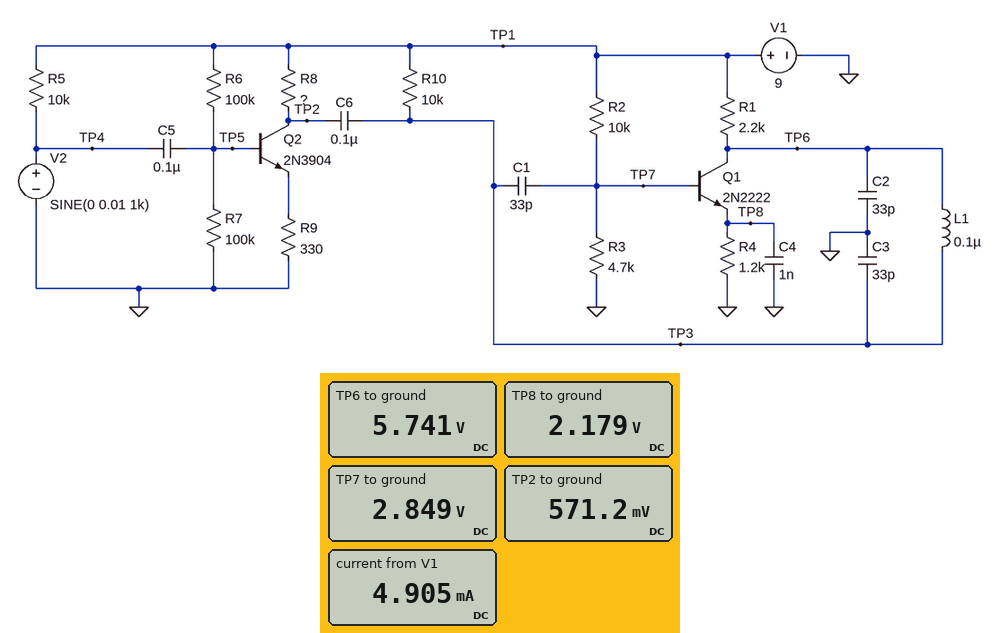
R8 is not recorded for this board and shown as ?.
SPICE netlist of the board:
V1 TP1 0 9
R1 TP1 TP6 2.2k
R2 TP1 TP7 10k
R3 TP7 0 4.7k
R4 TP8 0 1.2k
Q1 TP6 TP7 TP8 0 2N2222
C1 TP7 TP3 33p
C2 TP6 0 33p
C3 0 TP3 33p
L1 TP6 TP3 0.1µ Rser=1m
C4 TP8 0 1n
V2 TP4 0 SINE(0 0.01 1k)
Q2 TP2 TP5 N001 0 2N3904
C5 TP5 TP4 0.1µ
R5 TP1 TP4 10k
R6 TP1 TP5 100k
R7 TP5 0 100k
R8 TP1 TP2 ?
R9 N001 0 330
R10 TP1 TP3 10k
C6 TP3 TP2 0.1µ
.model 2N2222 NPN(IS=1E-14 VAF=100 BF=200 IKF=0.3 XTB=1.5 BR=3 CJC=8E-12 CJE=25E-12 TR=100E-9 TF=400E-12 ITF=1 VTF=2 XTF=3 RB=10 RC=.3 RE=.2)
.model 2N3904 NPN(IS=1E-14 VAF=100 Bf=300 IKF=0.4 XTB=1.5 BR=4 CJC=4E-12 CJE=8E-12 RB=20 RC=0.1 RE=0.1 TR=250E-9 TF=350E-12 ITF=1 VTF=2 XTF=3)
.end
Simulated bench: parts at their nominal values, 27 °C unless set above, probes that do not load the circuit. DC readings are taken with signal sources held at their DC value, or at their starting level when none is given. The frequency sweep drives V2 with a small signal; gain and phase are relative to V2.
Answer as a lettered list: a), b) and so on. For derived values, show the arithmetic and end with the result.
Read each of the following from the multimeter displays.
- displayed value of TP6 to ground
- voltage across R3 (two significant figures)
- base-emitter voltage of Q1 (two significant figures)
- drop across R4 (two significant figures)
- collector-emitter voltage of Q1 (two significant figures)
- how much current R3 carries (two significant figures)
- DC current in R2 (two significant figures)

a) 5.741 V
b) 2.849 V = 2.8 V
c) 2.849 V - 2.179 V = 670 mV
d) 2.179 V = 2.2 V
e) 5.741 V - 2.179 V = 3.6 V
f) (2.849 V) / 4.7 kΩ = 610 µA
g) (9 V - 2.849 V) / 10 kΩ = 620 µA
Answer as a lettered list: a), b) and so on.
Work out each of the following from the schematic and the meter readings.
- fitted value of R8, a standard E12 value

a) 5.6 kΩ
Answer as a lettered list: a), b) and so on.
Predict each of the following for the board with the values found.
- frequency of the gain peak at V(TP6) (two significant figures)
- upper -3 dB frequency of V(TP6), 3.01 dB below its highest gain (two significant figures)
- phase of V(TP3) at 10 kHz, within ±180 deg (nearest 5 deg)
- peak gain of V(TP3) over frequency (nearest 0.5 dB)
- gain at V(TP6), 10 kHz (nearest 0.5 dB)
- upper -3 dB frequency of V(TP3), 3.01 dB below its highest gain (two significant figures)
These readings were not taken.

a) 98 MHz
b) 110 MHz
c) 160 deg
d) 3.5 dB
e) -25.5 dB
f) 120 MHz
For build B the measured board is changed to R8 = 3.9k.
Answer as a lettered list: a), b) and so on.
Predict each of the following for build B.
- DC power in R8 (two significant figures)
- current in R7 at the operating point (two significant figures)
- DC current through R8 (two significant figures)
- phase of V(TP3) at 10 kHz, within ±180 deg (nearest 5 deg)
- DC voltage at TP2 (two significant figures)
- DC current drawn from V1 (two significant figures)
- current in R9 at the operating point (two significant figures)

a) 17 mW
b) 14 µA
c) 2.1 mA
d) -170 deg
e) 780 mV
f) 5.5 mA
g) 2.2 mA
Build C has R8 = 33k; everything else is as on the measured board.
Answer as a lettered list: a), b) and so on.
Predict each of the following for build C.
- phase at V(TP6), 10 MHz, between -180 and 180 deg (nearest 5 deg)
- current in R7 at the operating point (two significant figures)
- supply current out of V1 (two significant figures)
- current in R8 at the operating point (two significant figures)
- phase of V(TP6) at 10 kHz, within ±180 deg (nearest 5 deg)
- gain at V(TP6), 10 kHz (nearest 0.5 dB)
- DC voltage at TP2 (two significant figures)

a) -15 deg
b) 7.6 µA
c) 3.7 mA
d) 270 µA
e) 25 deg
f) -11.5 dB
g) 130 mV
